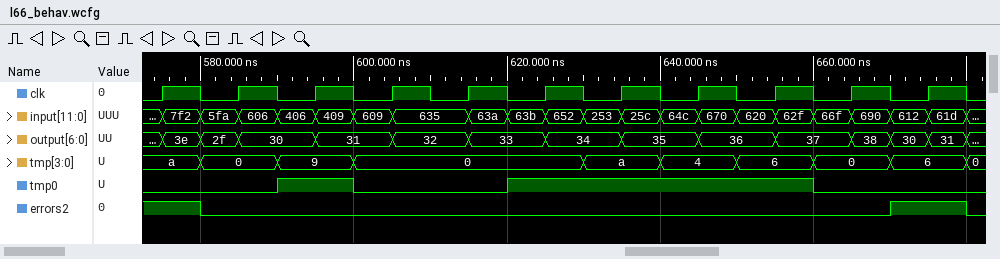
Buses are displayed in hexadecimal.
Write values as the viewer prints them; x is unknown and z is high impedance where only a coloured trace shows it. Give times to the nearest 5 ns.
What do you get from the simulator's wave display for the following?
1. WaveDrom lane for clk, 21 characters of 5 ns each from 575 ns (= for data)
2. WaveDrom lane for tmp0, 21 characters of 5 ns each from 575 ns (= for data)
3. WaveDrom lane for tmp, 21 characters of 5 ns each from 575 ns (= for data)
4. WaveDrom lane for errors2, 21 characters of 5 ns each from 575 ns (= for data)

{name: 'clk', wave: '101010101010101010101'}
{name: 'tmp0', wave: '0..1.0...1.......0...'}
{name: 'tmp', wave: '==.=.=.....=.=.=.=.=.', data: 'a 0 9 0 a 4 6 0 6'}
{name: 'errors2', wave: '10.................1.'}
